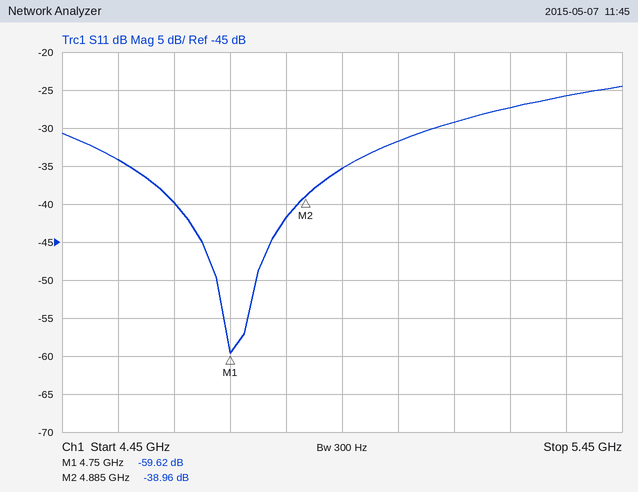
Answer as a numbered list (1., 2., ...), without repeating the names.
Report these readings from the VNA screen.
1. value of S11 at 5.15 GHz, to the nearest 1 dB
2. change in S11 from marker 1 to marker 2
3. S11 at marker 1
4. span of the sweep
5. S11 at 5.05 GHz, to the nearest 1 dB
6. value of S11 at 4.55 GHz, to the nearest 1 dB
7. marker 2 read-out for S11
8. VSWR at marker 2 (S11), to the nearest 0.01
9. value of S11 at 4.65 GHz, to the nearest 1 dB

1. -29 dB
2. 20.66 dB
3. -59.62 dB
4. 1 GHz
5. -32 dB
6. -34 dB
7. -38.96 dB
8. 1.02
9. -40 dB
